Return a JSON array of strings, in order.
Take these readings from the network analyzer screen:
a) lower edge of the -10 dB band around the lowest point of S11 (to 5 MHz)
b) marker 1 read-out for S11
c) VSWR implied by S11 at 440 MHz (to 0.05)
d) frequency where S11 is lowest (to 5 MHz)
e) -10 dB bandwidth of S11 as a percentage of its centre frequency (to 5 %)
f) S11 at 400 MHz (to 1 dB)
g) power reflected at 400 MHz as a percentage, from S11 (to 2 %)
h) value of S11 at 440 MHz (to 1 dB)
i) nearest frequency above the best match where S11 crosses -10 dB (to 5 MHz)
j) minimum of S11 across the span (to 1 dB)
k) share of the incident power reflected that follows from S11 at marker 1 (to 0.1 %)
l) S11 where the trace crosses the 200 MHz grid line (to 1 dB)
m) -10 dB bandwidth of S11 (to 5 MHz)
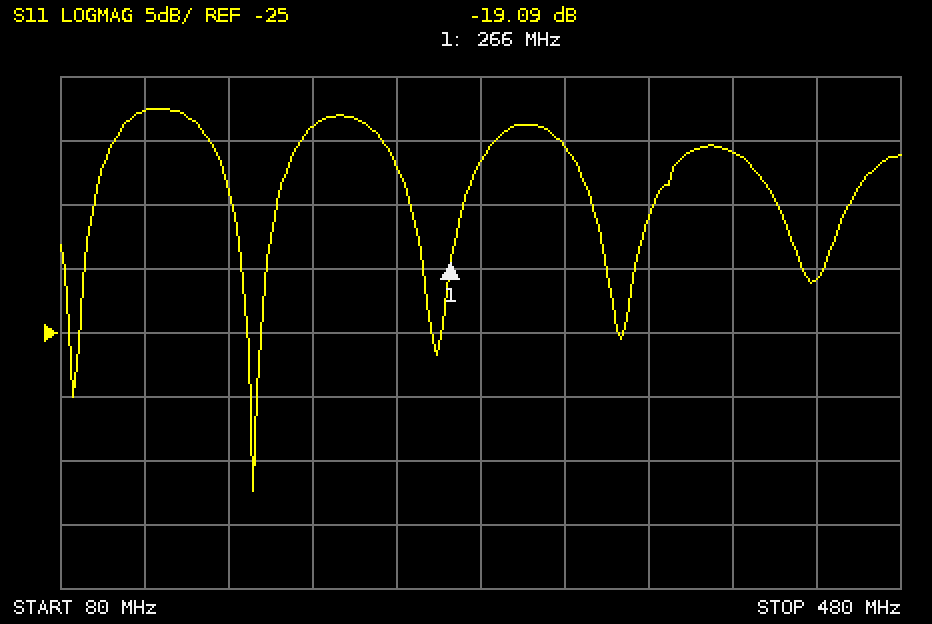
["150 MHz", "-19.09 dB", "1.20", "170 MHz", "25 %", "-11 dB", "8 %", "-21 dB", "195 MHz", "-37 dB", "1.2 %", "-9 dB", "45 MHz"]
